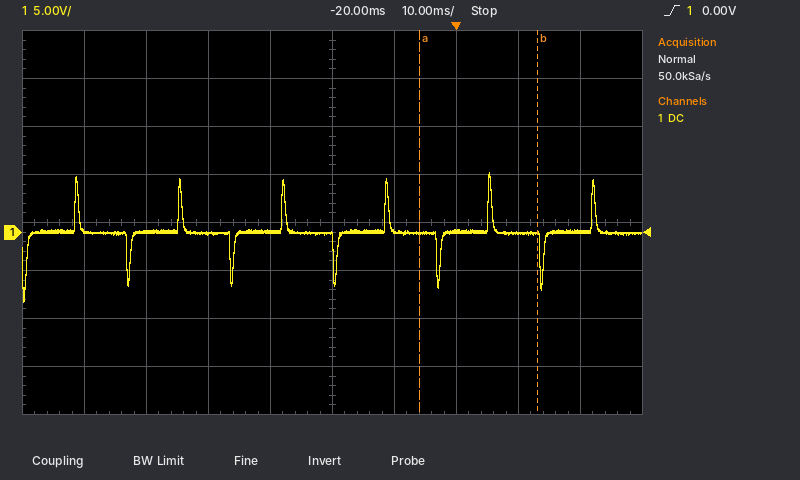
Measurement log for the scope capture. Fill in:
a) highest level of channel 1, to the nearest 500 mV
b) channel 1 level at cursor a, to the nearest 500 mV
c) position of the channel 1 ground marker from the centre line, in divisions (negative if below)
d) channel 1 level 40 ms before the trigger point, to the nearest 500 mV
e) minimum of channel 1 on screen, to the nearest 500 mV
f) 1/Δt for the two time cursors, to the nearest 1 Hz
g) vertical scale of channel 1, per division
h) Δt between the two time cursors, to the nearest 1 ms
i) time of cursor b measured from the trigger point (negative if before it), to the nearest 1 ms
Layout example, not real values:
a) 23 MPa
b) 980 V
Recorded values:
a) 6.0 V
b) 0.0 V
c) -0.2 div
d) 0.0 V
e) -7.0 V
f) 53 Hz
g) 5 V
h) 19 ms
i) +13 ms
